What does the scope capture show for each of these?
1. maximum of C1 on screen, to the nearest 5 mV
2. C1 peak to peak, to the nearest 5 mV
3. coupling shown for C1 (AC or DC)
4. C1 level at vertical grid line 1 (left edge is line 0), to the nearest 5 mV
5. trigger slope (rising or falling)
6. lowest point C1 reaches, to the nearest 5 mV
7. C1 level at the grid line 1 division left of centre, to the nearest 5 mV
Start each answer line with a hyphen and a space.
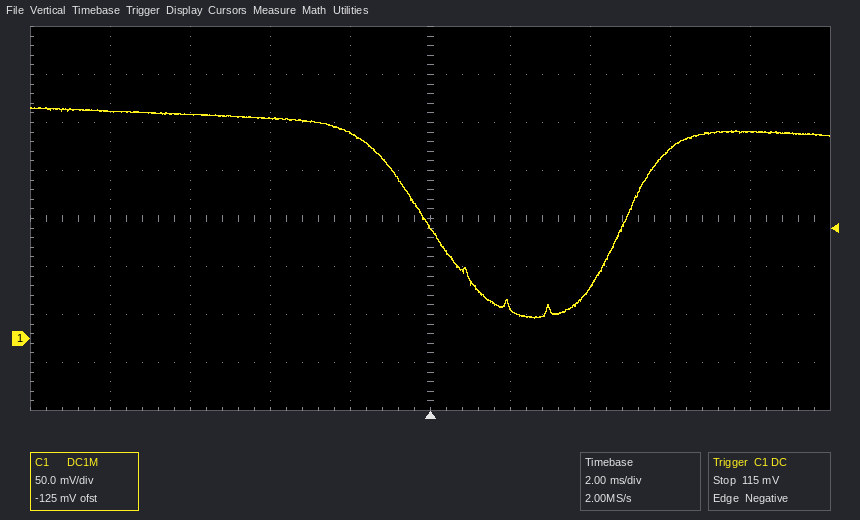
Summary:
- 240 mV
- 220 mV
- DC
- 235 mV
- falling
- 20 mV
- 215 mV
